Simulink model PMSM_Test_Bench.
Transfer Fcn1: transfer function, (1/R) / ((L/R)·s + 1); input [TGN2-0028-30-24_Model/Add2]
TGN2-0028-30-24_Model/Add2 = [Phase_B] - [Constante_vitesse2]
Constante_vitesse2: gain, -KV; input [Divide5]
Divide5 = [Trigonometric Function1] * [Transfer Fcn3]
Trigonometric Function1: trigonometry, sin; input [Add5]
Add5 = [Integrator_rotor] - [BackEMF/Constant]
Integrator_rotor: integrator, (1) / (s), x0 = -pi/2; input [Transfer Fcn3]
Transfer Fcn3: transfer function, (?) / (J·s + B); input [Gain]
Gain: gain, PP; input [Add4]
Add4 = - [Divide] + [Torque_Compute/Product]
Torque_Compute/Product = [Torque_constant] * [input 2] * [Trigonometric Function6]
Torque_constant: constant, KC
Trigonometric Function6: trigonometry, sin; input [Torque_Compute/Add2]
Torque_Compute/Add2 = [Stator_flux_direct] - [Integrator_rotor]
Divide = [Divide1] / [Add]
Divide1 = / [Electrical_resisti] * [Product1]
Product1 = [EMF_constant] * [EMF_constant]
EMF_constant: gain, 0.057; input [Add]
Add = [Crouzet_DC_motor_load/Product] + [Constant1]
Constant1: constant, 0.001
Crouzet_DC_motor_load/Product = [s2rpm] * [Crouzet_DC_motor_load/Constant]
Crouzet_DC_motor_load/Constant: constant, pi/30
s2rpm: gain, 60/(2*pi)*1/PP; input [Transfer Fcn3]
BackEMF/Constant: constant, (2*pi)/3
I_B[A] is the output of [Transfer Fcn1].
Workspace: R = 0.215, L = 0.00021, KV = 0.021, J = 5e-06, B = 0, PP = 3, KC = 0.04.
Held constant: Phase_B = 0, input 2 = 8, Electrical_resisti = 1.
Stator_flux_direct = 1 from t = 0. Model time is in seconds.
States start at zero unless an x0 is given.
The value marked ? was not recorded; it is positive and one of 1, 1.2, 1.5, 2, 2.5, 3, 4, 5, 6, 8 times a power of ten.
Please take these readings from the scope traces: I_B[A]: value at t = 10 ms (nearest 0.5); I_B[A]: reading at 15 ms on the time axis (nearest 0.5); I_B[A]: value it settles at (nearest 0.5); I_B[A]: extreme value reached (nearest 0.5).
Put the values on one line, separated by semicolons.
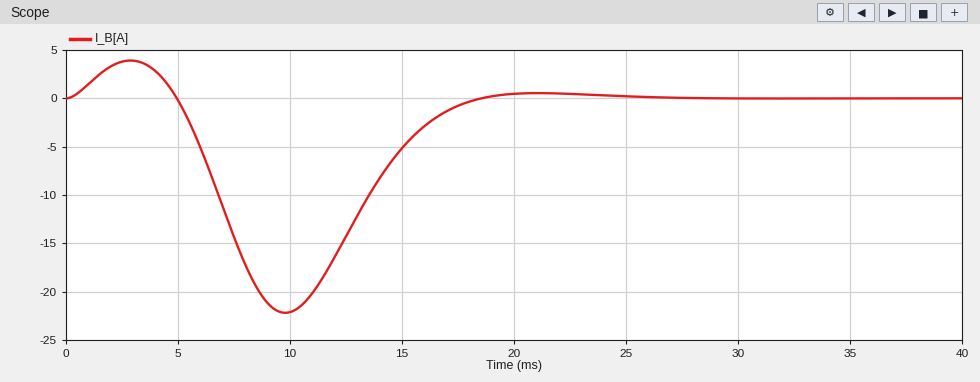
-22.0; -5.0; 0.0; -22.0
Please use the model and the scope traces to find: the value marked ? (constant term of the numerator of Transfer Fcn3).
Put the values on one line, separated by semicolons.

1
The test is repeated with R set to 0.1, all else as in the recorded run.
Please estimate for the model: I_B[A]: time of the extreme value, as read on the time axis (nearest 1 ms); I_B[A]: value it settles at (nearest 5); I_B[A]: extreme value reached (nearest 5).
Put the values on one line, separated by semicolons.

11 ms; 0; -40
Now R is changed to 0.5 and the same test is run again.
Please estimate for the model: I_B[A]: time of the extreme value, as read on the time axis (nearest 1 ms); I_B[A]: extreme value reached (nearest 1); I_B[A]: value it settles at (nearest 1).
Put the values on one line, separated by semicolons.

9 ms; -10; 0
